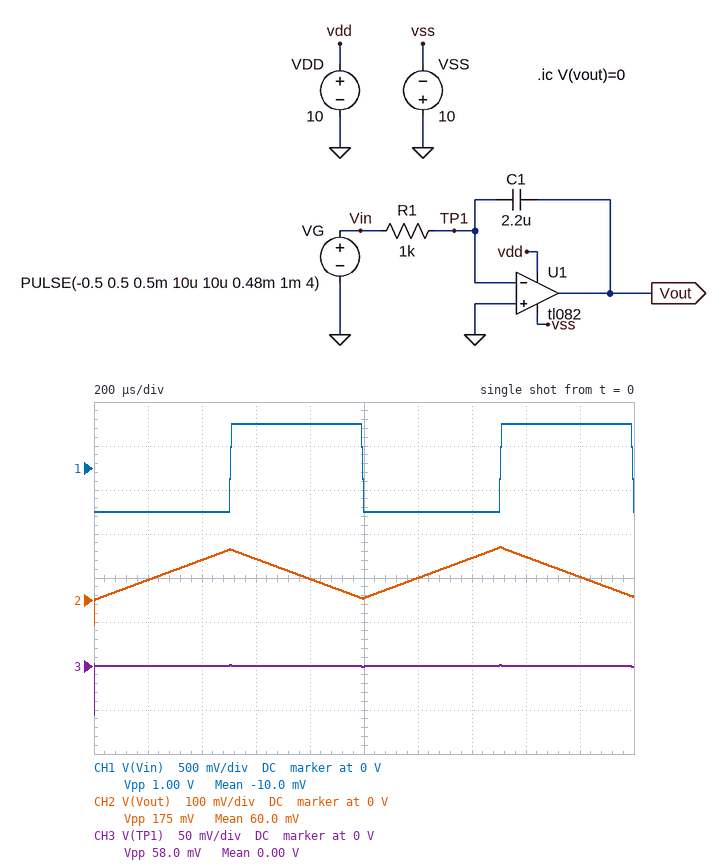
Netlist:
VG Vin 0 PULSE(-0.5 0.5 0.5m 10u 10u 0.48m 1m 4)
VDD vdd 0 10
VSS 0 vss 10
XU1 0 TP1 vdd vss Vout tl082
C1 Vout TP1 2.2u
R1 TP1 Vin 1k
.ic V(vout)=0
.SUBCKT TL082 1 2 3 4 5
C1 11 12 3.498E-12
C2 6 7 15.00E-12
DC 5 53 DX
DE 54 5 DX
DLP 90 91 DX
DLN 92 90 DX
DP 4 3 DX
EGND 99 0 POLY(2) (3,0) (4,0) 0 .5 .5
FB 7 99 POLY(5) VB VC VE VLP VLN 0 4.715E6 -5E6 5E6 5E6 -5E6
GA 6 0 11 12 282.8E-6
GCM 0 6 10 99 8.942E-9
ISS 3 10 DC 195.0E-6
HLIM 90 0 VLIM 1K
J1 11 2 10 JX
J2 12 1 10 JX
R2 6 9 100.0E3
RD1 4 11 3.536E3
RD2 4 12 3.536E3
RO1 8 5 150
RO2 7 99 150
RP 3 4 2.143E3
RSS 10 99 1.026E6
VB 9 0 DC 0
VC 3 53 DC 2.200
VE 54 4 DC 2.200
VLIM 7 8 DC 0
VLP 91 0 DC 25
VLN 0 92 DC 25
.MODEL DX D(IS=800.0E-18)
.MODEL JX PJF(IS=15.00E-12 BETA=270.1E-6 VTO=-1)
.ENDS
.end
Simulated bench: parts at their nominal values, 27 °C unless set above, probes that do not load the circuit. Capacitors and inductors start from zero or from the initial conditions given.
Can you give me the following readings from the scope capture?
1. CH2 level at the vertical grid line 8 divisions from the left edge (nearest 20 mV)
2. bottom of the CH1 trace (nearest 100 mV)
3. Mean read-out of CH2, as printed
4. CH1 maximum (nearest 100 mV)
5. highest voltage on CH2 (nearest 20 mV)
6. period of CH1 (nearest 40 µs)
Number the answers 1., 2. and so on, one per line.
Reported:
1. 100 mV
2. -500 mV
3. 60.0 mV
4. 500 mV
5. 120 mV
6. 1.00 ms
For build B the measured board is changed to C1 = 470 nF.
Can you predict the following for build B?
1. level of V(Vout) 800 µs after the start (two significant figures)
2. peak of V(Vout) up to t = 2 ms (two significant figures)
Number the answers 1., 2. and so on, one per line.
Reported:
1. 220 mV
2. 560 mV
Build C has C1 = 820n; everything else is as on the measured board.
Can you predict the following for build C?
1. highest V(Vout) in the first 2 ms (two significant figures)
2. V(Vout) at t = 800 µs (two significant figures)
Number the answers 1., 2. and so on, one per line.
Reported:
1. 320 mV
2. 130 mV
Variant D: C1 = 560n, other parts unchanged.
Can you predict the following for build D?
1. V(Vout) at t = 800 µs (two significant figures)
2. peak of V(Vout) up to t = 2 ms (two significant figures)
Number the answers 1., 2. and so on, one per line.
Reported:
1. 190 mV
2. 470 mV
